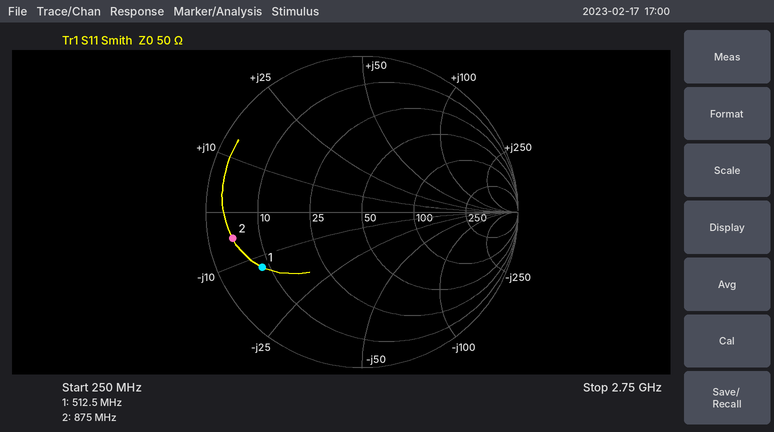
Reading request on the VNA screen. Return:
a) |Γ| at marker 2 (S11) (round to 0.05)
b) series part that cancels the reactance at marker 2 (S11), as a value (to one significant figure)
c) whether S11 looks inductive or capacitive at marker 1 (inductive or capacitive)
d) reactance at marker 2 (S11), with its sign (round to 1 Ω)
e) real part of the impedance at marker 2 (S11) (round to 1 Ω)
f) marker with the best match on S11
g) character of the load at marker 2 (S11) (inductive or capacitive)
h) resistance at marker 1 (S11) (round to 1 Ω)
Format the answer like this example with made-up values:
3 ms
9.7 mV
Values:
0.85
900 pH
capacitive
-5 Ω
4 Ω
marker 1
capacitive
8 Ω
